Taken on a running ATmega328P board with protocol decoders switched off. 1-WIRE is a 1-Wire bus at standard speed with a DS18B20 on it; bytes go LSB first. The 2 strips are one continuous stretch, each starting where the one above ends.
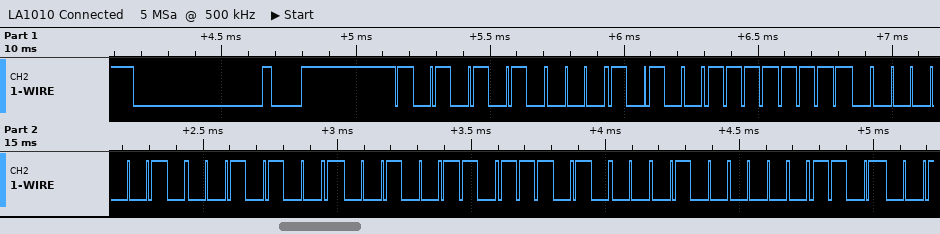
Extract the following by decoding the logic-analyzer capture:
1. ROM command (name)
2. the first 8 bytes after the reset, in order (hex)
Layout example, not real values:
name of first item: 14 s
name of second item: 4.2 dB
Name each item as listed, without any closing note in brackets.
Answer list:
ROM command: Match ROM
the first 8 bytes after the reset, in order: 55 28 FF 40 94 64 17 02
